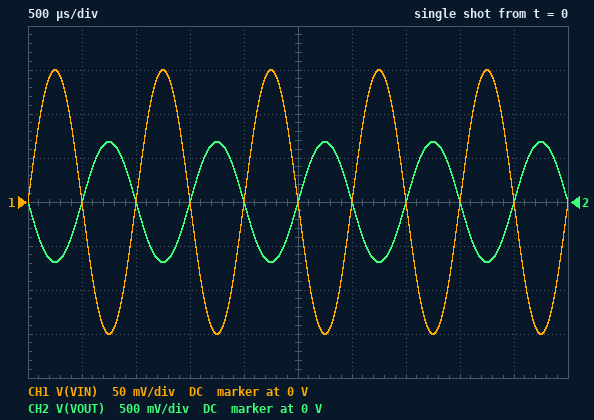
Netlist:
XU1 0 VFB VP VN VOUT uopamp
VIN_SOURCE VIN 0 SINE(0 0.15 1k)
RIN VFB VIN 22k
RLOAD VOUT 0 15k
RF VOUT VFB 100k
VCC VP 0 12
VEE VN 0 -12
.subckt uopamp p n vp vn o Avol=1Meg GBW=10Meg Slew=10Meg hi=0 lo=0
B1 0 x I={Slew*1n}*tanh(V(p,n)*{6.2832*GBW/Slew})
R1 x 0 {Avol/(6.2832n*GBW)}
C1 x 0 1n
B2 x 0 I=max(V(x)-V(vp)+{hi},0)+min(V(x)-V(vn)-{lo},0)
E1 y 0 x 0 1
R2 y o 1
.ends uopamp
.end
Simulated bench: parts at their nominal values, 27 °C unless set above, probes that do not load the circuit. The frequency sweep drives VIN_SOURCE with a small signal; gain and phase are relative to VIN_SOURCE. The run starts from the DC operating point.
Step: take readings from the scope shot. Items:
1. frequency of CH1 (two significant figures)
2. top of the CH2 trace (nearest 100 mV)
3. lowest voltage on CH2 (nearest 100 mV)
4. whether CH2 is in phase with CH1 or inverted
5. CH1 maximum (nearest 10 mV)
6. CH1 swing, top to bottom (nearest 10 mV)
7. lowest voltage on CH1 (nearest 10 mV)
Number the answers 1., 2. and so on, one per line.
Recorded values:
1. 1.0 kHz
2. 700 mV
3. -700 mV
4. inverted
5. 150 mV
6. 300 mV
7. -150 mV
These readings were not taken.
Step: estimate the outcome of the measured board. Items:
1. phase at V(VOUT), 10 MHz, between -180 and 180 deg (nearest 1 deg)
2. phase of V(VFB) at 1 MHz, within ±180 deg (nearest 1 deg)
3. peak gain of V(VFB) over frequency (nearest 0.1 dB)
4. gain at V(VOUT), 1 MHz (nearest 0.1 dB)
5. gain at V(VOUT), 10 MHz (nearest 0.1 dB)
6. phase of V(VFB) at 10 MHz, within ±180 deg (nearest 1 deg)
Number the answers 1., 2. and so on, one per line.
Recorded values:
1. 100 deg
2. 61 deg
3. -1.7 dB
4. 12.0 dB
5. -1.9 dB
6. 10 deg
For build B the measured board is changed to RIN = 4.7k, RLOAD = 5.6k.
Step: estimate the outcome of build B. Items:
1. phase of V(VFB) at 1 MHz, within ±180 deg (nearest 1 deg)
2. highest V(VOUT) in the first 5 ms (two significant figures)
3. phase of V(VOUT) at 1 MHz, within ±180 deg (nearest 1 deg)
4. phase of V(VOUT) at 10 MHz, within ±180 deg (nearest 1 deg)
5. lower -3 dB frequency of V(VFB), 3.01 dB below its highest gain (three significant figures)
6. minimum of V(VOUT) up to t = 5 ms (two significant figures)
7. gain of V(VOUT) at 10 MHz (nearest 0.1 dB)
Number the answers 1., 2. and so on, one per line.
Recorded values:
1. 24 deg
2. 3.2 V
3. 114 deg
4. 93 deg
5. 449 kHz
6. -3.2 V
7. -0.4 dB
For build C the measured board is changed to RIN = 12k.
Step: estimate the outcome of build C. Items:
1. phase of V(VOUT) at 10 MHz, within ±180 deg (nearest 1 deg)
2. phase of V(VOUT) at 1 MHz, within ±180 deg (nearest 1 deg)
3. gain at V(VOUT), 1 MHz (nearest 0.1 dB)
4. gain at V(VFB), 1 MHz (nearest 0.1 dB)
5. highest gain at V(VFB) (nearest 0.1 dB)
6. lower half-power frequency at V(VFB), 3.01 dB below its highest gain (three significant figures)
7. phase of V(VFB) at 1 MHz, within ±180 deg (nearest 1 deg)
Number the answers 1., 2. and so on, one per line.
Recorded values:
1. 96 deg
2. 137 deg
3. 15.7 dB
4. -4.3 dB
5. -1.0 dB
6. 1.07 MHz
7. 47 deg
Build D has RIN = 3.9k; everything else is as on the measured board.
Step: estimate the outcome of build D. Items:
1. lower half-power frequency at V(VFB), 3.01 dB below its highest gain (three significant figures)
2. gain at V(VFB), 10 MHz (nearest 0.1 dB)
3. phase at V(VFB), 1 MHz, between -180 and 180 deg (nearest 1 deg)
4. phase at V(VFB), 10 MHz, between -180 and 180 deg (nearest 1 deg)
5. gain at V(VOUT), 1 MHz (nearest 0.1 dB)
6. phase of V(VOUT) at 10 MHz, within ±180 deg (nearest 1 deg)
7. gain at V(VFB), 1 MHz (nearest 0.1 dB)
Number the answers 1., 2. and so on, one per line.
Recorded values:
1. 375 kHz
2. -0.3 dB
3. 21 deg
4. 2 deg
5. 19.1 dB
6. 92 deg
7. -0.9 dB
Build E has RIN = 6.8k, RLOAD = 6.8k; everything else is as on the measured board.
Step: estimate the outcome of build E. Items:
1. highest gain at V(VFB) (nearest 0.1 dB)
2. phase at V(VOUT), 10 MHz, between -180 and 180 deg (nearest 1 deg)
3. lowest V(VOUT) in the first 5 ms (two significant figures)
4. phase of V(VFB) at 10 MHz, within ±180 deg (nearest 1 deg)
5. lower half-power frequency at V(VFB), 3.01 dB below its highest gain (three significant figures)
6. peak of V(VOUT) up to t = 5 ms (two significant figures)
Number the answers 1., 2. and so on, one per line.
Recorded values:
1. -0.6 dB
2. 94 deg
3. -2.2 V
4. 4 deg
5. 637 kHz
6. 2.2 V
